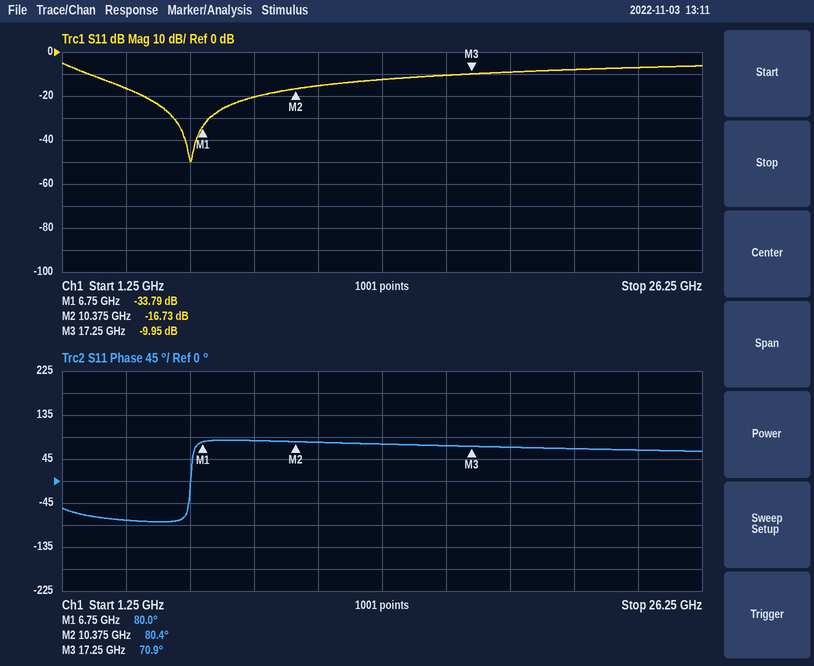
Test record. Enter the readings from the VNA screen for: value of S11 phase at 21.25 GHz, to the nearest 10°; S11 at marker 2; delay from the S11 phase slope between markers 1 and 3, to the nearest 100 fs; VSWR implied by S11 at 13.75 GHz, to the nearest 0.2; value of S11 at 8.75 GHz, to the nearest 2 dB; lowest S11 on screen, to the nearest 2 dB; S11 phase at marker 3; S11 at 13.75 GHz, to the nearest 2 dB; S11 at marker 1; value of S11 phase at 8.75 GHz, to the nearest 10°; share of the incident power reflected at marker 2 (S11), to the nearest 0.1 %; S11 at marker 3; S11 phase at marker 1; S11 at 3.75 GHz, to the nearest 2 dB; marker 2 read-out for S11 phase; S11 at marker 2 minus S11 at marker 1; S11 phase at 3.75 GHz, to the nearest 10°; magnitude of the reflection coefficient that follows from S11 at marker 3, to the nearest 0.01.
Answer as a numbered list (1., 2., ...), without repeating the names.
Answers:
1. 70°
2. -16.73 dB
3. 2.4 ps
4. 1.6
5. -20 dB
6. -50 dB
7. 70.9°
8. -12 dB
9. -33.79 dB
10. 80°
11. 2.1 %
12. -9.95 dB
13. 80.0°
14. -16 dB
15. 80.4°
16. 17.06 dB
17. -80°
18. 0.32
